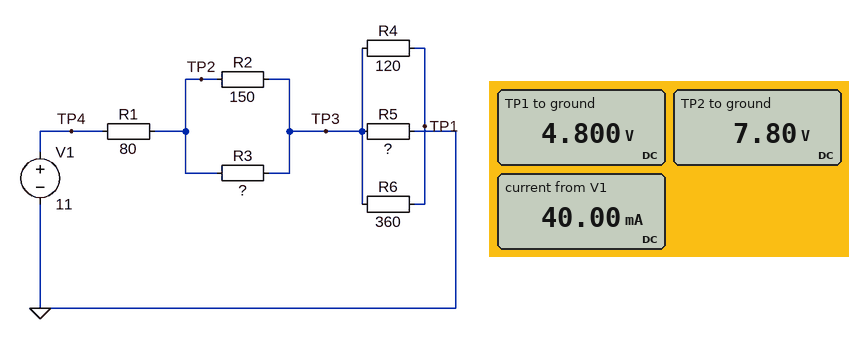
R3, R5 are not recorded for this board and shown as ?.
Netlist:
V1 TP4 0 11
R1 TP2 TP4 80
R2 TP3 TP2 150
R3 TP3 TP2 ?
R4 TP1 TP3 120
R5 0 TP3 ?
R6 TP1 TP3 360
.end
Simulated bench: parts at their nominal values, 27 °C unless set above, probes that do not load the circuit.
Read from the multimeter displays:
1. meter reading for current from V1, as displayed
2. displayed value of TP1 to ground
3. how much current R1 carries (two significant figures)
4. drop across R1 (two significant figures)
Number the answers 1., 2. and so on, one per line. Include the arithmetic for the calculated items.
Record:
1. 40.00 mA
2. 4.800 V
3. (11 V - 7.8 V) / 80 Ω = 40 mA
4. 11 V - 7.8 V = 3.2 V
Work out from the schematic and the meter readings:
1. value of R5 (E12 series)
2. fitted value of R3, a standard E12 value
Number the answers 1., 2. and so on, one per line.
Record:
1. 120 Ω
2. 150 Ω
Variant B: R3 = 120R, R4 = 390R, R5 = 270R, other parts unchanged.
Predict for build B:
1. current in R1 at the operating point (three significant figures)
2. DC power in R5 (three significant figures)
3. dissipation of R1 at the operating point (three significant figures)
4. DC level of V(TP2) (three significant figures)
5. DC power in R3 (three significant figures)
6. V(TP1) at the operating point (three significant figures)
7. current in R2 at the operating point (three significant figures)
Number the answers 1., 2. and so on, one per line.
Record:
1. 26.4 mA
2. 188 mW
3. 55.8 mW
4. 8.89 V
5. 25.8 mW
6. 7.13 V
7. 11.7 mA
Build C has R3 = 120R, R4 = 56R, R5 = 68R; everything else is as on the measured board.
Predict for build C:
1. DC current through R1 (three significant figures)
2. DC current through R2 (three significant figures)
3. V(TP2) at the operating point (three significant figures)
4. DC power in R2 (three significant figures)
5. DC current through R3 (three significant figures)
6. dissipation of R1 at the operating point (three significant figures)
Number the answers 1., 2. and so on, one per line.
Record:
1. 51.2 mA
2. 22.8 mA
3. 6.90 V
4. 77.8 mW
5. 28.5 mA
6. 210 mW
